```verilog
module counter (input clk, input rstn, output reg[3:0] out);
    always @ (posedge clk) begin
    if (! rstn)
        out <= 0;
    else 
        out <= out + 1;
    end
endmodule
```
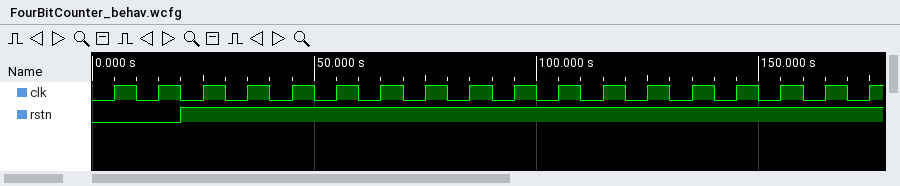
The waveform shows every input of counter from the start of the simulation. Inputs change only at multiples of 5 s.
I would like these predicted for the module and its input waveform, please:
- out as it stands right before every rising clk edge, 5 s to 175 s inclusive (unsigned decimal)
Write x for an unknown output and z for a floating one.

x, 0, 0, 1, 2, 3, 4, 5, 6, 7, 8, 9, 10, 11, 12, 13, 14, 15
